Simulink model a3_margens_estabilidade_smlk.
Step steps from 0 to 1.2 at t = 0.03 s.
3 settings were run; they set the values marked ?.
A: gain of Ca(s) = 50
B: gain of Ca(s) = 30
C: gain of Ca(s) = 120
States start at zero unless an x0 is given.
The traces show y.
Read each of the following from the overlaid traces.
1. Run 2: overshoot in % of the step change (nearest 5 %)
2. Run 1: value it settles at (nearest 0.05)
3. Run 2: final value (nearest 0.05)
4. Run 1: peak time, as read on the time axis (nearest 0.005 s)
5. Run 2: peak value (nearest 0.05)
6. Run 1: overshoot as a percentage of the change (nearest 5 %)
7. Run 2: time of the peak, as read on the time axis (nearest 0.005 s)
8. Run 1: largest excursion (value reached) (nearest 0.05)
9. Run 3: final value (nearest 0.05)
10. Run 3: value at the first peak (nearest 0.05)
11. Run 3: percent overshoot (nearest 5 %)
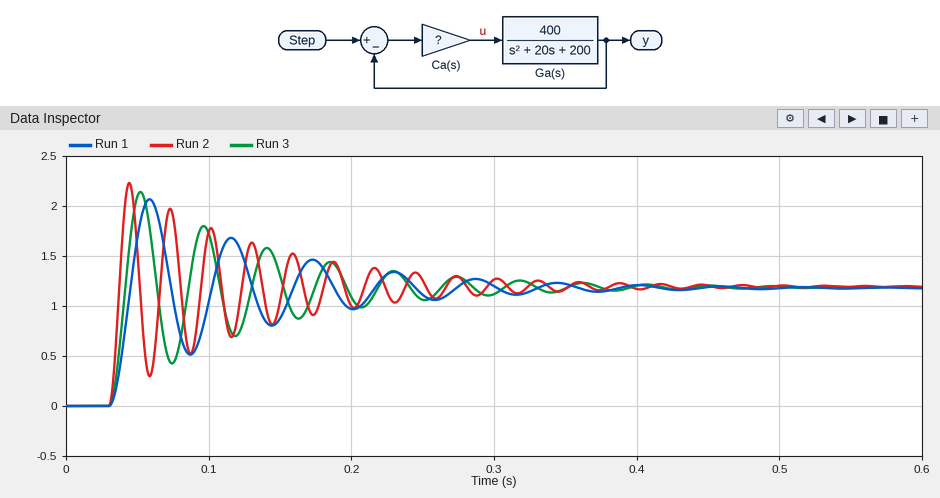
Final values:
85 %
1.20
1.20
0.060 s
2.25
75 %
0.045 s
2.05
1.20
2.15
80 %
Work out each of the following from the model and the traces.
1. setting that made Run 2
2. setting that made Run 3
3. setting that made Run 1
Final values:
C
A
B
